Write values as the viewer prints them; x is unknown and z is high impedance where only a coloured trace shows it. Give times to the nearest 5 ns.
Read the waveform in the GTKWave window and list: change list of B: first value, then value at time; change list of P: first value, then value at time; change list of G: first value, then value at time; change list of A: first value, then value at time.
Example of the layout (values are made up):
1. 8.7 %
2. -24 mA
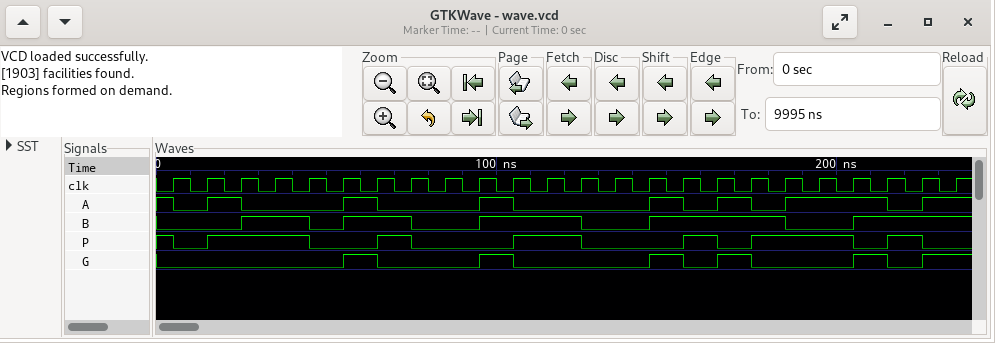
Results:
1. 0, 1 at 25 ns, 0 at 45 ns, 1 at 55 ns, 0 at 75 ns, 1 at 95 ns, 0 at 125 ns, 1 at 145 ns, 0 at 185 ns, 1 at 205 ns
2. 1, 0 at 5 ns, 1 at 15 ns, 0 at 45 ns, 1 at 65 ns, 0 at 75 ns, 1 at 105 ns, 0 at 125 ns, 1 at 155 ns, 0 at 165 ns, 1 at 175 ns, 0 at 205 ns, 1 at 215 ns, 0 at 225 ns
3. 0, 1 at 55 ns, 0 at 65 ns, 1 at 95 ns, 0 at 105 ns, 1 at 145 ns, 0 at 155 ns, 1 at 165 ns, 0 at 175 ns, 1 at 205 ns, 0 at 215 ns, 1 at 225 ns
4. 1, 0 at 5 ns, 1 at 15 ns, 0 at 25 ns, 1 at 55 ns, 0 at 65 ns, 1 at 95 ns, 0 at 105 ns, 1 at 145 ns, 0 at 155 ns, 1 at 165 ns, 0 at 175 ns, 1 at 185 ns, 0 at 215 ns, 1 at 225 ns
